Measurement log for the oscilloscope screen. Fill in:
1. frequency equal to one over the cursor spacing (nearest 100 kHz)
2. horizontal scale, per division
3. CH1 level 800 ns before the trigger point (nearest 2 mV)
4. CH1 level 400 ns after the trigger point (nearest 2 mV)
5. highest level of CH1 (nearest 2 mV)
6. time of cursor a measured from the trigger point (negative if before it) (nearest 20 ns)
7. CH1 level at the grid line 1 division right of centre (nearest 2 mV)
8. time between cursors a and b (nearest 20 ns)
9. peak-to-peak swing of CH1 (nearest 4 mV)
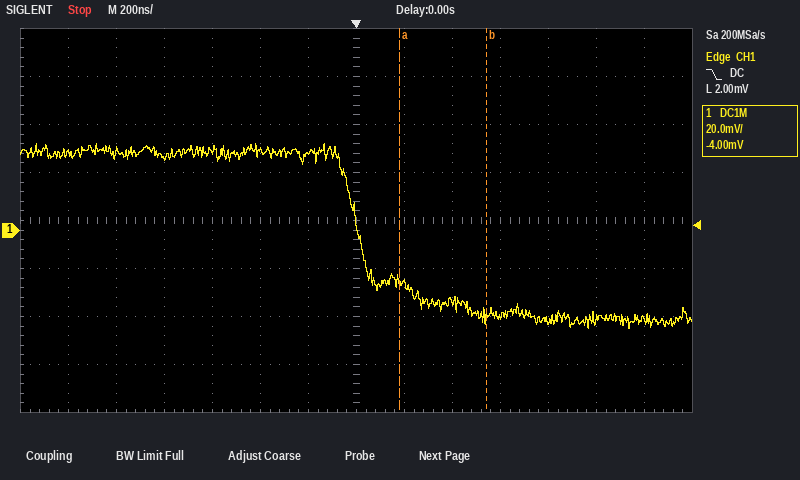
2.8 MHz
200 ns
30 mV
-30 mV
36 mV
+180 ns
-22 mV
360 ns
76 mV
